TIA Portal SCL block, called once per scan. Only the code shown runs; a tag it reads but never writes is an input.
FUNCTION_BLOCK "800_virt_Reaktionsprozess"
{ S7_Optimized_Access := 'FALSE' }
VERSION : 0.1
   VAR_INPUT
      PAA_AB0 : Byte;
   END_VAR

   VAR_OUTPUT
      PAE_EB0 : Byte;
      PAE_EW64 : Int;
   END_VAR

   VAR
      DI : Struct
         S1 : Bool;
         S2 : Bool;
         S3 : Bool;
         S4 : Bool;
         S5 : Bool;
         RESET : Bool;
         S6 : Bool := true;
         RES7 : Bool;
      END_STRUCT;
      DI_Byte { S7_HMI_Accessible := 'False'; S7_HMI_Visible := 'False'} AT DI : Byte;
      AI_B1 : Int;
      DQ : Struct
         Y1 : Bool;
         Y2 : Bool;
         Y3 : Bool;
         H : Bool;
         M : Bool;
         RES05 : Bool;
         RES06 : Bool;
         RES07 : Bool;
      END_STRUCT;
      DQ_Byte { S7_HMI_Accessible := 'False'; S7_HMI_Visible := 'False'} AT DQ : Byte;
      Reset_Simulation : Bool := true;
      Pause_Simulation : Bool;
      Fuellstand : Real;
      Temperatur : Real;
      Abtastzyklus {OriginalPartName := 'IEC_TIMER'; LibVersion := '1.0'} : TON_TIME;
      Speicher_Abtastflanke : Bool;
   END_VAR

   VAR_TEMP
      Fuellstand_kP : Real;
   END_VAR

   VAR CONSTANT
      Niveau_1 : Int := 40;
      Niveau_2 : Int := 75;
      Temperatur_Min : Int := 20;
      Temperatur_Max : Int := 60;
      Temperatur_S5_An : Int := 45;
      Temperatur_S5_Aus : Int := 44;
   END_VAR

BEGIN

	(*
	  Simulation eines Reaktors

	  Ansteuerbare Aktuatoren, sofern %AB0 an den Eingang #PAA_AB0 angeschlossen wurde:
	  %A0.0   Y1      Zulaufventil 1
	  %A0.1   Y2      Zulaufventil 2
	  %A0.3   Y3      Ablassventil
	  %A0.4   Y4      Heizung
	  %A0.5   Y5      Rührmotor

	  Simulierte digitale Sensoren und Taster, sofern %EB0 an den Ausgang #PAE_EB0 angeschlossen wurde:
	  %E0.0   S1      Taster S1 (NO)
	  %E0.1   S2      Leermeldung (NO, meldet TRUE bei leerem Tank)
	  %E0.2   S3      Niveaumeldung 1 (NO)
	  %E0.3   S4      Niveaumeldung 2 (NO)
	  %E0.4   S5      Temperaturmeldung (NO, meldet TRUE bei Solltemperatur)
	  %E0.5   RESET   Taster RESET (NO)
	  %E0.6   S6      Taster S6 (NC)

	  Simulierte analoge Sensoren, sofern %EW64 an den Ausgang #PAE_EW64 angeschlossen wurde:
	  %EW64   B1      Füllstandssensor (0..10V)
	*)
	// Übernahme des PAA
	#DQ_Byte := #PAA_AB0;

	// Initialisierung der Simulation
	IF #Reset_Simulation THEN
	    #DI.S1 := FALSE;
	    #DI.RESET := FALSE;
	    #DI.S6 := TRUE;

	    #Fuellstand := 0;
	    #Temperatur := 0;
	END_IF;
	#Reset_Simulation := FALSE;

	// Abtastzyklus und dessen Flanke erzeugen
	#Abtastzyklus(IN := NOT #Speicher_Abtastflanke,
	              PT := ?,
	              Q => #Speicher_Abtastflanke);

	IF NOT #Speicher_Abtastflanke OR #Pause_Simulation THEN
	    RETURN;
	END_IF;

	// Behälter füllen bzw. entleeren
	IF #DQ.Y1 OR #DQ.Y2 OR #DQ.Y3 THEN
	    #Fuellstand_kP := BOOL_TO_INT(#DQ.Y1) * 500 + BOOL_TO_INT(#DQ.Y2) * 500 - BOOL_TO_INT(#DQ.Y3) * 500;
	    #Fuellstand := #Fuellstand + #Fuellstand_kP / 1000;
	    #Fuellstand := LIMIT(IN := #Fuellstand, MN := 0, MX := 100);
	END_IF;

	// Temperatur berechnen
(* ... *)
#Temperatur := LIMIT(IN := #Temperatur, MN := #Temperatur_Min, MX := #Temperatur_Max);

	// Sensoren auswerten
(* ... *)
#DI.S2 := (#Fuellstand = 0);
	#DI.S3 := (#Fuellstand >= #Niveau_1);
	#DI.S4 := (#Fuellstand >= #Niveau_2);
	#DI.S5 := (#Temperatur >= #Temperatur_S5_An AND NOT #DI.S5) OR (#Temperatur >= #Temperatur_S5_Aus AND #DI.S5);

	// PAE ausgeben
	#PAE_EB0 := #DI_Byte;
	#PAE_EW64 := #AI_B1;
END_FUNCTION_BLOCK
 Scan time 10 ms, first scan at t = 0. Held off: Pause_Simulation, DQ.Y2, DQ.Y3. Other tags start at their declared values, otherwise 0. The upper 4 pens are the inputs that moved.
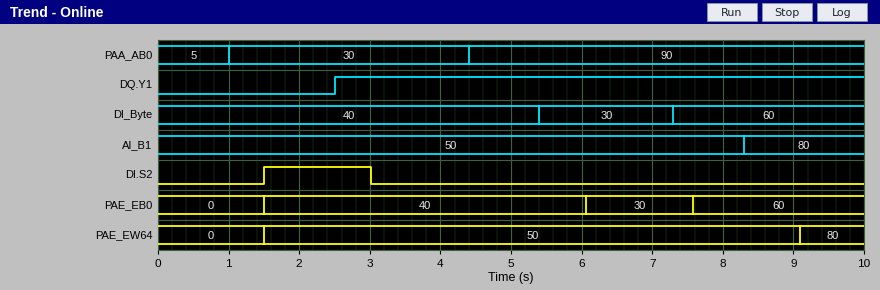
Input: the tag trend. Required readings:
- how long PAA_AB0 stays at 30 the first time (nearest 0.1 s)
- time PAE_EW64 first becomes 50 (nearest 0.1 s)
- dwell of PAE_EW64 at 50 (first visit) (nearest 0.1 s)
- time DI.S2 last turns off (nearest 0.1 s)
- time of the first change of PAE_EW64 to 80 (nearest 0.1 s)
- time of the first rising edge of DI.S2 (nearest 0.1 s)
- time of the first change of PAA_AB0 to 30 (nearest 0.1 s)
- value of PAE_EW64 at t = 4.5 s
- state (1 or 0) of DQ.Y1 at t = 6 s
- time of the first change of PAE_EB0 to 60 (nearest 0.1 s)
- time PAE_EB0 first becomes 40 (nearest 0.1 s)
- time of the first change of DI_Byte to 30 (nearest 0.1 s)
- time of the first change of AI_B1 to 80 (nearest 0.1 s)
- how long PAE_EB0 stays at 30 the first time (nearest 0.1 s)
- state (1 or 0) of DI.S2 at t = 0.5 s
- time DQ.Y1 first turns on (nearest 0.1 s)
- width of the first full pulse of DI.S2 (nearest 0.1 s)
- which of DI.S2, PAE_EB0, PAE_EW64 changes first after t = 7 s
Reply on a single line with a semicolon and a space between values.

3.4 s; 1.5 s; 7.6 s; 3.0 s; 9.1 s; 1.5 s; 1.0 s; 50; 1; 7.6 s; 1.5 s; 5.4 s; 8.3 s; 1.5 s; 0; 2.5 s; 1.5 s; PAE_EB0
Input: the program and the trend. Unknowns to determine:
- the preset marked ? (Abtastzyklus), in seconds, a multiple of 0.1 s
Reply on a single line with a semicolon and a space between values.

1.5 s
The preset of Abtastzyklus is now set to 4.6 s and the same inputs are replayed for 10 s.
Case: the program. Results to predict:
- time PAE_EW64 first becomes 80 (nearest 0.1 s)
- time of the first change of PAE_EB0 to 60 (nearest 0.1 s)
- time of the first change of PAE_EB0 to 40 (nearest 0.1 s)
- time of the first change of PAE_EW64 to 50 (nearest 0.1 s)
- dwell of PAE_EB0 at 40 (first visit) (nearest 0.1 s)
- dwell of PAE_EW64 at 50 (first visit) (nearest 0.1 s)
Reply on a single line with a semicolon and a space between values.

9.2 s; 9.2 s; 4.6 s; 4.6 s; 4.6 s; 4.6 s
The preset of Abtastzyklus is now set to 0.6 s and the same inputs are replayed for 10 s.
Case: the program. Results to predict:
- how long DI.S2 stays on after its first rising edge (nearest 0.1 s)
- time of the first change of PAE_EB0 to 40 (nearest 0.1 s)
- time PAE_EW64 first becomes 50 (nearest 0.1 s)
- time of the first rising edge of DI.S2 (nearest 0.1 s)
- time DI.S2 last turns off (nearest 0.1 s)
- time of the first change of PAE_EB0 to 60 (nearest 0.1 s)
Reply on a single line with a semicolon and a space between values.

2.5 s; 0.6 s; 0.6 s; 0.6 s; 3.1 s; 7.4 s
